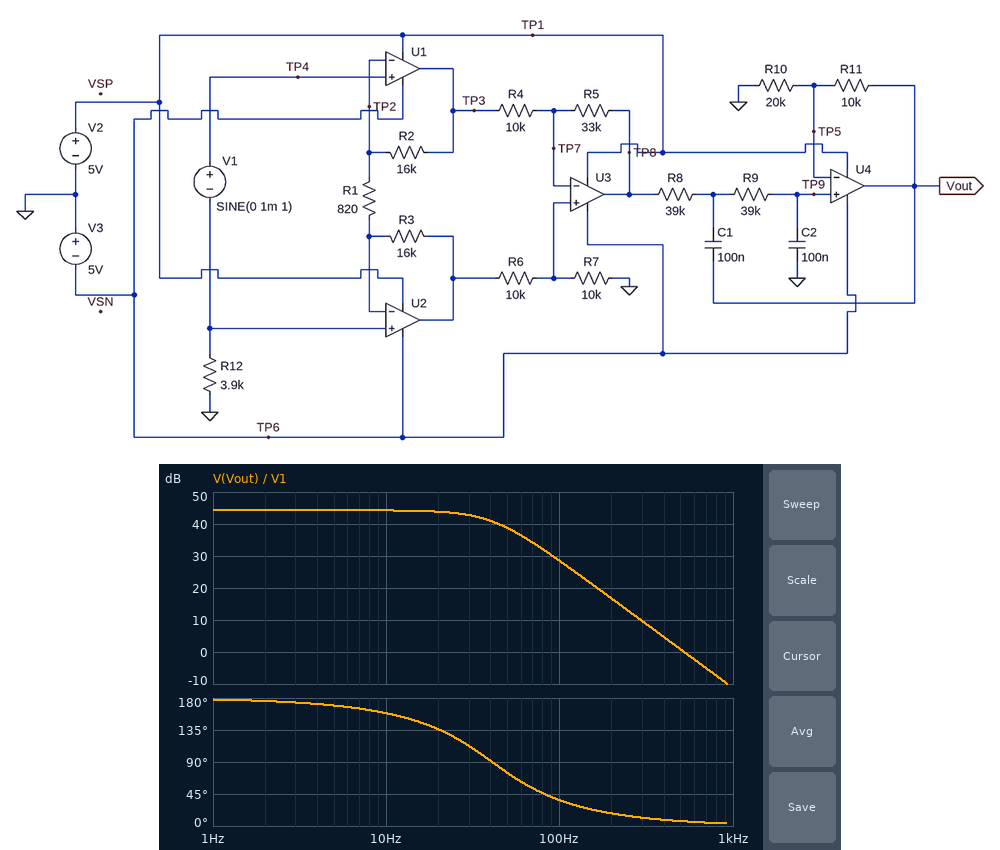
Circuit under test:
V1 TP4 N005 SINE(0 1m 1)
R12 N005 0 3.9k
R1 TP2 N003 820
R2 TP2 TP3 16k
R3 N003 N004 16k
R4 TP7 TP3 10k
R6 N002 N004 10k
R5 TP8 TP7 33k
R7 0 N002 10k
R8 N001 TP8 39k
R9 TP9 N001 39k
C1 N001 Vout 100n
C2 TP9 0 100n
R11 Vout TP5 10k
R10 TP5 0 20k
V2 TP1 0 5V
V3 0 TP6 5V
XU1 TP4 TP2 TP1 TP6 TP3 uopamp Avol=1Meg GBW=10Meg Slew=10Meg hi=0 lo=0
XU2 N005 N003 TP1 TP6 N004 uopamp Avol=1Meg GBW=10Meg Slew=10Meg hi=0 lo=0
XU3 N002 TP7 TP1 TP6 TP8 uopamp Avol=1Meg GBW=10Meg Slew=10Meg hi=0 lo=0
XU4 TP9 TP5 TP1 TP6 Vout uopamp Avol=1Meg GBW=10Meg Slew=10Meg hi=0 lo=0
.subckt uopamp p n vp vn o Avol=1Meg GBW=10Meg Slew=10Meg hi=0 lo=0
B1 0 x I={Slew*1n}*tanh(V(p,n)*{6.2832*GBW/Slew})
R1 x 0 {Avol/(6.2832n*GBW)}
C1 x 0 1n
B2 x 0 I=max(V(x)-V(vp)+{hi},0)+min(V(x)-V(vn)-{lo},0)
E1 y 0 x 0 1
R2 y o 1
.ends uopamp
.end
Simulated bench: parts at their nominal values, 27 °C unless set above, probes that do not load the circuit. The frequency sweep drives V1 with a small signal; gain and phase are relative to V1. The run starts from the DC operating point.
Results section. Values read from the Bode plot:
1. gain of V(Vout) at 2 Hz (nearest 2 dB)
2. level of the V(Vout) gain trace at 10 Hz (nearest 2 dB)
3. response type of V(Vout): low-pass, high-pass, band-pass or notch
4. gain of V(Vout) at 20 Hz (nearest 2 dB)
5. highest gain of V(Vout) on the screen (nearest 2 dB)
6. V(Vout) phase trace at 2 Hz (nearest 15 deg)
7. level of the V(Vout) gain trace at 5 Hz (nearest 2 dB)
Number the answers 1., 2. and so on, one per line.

1. 44 dB
2. 44 dB
3. low-pass
4. 44 dB
5. 44 dB
6. 180 deg
7. 44 dB
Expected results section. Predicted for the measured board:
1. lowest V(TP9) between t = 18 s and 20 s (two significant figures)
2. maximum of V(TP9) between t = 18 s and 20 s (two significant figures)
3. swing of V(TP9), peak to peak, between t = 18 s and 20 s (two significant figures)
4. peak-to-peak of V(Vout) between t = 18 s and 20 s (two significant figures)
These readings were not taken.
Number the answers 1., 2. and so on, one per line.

1. -110 mV
2. 110 mV
3. 220 mV
4. 330 mV
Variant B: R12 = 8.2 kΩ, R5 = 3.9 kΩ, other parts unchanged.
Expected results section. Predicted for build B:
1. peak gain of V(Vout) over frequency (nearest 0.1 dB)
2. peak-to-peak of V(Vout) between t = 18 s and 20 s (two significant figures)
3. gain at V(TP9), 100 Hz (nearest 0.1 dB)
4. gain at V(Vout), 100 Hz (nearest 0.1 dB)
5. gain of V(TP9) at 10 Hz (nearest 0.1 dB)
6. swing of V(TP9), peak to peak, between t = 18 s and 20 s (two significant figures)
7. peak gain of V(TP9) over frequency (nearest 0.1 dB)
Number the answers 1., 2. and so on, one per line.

1. 30.2 dB
2. 65 mV
3. 10.8 dB
4. 14.3 dB
5. 26.6 dB
6. 43 mV
7. 26.7 dB
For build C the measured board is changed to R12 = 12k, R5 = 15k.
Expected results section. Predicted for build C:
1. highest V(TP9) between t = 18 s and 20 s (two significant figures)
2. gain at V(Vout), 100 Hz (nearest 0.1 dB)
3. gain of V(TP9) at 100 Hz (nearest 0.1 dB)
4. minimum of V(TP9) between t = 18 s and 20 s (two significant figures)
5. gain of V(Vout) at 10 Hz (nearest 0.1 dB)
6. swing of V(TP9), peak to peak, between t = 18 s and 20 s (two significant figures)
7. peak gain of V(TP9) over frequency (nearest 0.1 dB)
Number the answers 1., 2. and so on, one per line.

1. 55 mV
2. 22.5 dB
3. 19.0 dB
4. -55 mV
5. 38.3 dB
6. 110 mV
7. 34.8 dB
